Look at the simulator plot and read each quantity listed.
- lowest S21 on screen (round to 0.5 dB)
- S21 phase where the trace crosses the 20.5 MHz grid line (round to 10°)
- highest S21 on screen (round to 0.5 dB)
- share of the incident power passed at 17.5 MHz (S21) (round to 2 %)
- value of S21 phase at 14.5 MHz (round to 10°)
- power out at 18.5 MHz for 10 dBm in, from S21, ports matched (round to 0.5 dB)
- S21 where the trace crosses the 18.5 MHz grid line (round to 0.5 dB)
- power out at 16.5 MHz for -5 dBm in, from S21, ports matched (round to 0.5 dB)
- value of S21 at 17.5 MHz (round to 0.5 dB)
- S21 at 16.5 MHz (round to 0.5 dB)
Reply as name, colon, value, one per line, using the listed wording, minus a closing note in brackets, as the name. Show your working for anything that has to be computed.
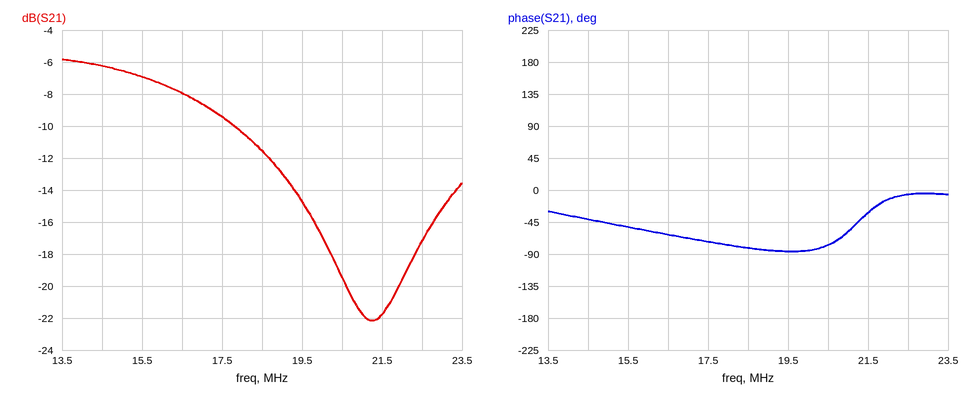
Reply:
lowest S21 on screen: -22.0 dB
S21 phase where the trace crosses the 20.5 MHz grid line: -80°
highest S21 on screen: -6.0 dB
share of the incident power passed at 17.5 MHz (S21): 10^(-9.5/10) ≈ 11.2 %, so 12 % to the nearest 2 %
value of S21 phase at 14.5 MHz: -40°
power out at 18.5 MHz for 10 dBm in, from S21, ports matched: 10 dBm + (-11.5 dB) = -1.5 dBm
S21 where the trace crosses the 18.5 MHz grid line: -11.5 dB
power out at 16.5 MHz for -5 dBm in, from S21, ports matched: -5 dBm + (-8.0 dB) = -13.0 dBm
value of S21 at 17.5 MHz: -9.5 dB
S21 at 16.5 MHz: -8.0 dB
